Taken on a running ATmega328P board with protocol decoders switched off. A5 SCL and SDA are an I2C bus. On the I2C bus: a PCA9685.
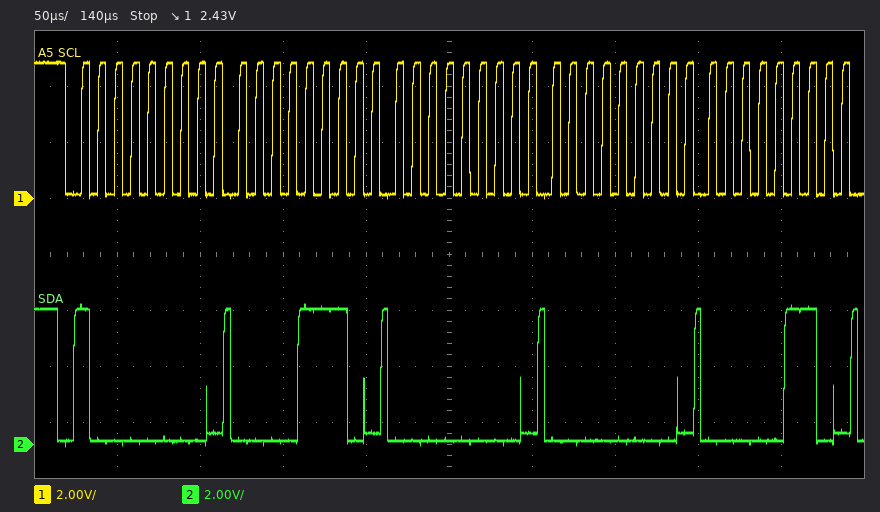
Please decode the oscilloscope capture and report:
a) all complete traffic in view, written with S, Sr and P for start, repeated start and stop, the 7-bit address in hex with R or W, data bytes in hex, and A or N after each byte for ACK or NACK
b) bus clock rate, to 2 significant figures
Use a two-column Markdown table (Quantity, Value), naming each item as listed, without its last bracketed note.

| Quantity | Value |
|---|---|
| all complete traffic in view, written with S, Sr and P for start, repeated start and stop, the 7-bit address in hex with R or W, data bytes in hex, and A or N after each byte for ACK or NACK | S 40W A 0E A 00 A 00 A 06 A |
| bus clock rate, to 2 significant figures | 100 kHz |
